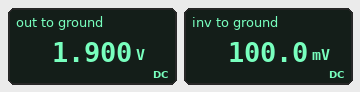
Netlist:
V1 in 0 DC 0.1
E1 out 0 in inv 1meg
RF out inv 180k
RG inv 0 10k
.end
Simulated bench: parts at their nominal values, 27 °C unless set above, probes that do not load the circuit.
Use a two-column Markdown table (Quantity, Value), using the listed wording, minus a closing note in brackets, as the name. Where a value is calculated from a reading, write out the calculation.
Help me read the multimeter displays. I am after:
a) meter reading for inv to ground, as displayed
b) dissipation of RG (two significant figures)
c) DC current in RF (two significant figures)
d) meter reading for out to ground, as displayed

| Quantity | Value |
|---|---|
| meter reading for inv to ground, as displayed | 100.0 mV |
| dissipation of RG | (100 mV)^2 / 10 kΩ = 1.0 µW |
| DC current in RF | (1.9 V - 100 mV) / 180 kΩ = 10 µA |
| meter reading for out to ground, as displayed | 1.900 V |
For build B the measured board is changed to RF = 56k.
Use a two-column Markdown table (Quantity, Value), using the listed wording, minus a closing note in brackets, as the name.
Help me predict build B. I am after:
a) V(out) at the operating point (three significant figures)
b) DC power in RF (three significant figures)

| Quantity | Value |
|---|---|
| V(out) at the operating point | 660 mV |
| DC power in RF | 5.60 µW |
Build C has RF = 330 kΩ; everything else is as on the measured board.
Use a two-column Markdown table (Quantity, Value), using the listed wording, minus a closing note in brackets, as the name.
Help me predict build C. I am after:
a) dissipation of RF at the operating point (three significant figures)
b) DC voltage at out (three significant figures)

| Quantity | Value |
|---|---|
| dissipation of RF at the operating point | 33.0 µW |
| DC voltage at out | 3.40 V |
